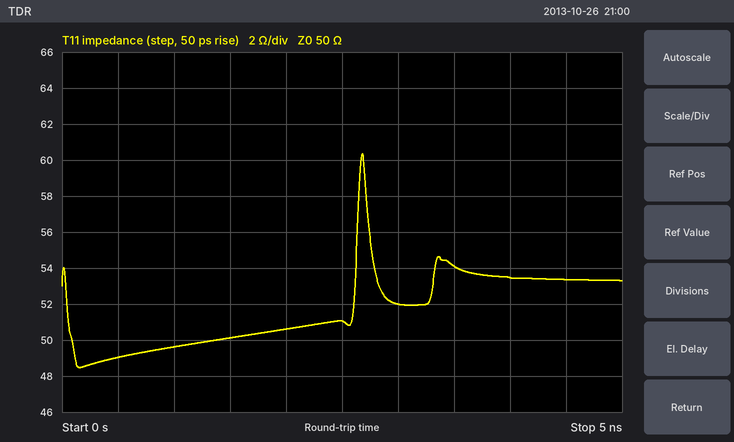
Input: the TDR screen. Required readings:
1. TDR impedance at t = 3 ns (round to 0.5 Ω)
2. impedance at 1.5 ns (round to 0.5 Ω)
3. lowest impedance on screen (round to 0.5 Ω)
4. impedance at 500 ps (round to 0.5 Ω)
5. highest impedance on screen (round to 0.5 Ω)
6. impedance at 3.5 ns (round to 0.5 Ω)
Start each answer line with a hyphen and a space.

- 52.0 Ω
- 50.0 Ω
- 48.5 Ω
- 49.0 Ω
- 60.5 Ω
- 54.0 Ω
